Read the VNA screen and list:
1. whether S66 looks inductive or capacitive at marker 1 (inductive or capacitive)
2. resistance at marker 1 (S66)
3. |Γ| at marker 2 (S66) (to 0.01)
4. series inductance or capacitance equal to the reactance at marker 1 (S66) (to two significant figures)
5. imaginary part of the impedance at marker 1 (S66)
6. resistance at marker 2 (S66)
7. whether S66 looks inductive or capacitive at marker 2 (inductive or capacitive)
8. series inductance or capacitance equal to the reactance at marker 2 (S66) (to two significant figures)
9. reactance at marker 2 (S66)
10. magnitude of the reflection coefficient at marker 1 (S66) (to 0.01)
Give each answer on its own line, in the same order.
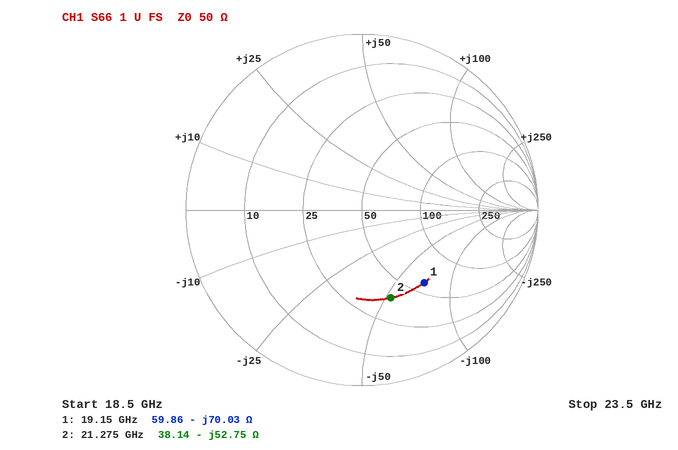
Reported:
capacitive
59.86 Ω
0.53
120 fF
-70.03 Ω
38.14 Ω
capacitive
140 fF
-52.75 Ω
0.54
